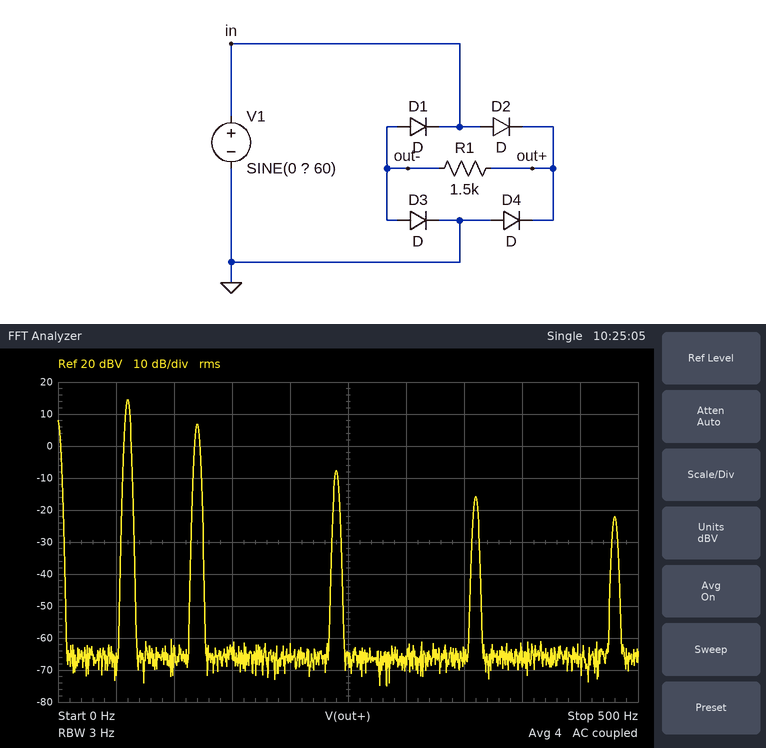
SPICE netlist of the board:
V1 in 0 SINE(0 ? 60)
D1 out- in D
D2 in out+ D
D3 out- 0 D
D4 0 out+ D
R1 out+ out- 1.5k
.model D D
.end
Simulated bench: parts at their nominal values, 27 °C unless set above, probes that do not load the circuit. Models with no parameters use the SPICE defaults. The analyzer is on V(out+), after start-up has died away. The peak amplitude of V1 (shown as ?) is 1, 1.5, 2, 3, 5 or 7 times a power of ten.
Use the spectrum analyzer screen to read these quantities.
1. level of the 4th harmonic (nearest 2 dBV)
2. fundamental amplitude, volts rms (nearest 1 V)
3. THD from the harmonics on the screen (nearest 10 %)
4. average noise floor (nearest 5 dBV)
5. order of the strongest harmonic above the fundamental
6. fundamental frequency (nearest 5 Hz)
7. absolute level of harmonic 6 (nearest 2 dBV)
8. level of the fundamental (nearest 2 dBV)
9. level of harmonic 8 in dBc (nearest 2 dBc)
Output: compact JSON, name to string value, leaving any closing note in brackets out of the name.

{"level of the 4th harmonic": "-8 dBV", "fundamental amplitude, volts rms": "5 V", "THD from the harmonics on the screen": "40 %", "average noise floor": "-65 dBV", "order of the strongest harmonic above the fundamental": "2", "fundamental frequency": "60 Hz", "absolute level of harmonic 6": "-16 dBV", "level of the fundamental": "14 dBV", "level of harmonic 8 in dBc": "-36 dBc"}
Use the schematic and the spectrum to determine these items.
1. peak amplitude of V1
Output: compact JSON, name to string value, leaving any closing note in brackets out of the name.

{"peak amplitude of V1": "15 V"}
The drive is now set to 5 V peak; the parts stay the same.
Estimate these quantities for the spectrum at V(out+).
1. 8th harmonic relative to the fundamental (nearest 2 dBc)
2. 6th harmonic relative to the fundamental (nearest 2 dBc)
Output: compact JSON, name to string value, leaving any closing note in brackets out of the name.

{"8th harmonic relative to the fundamental": "-44 dBc", "6th harmonic relative to the fundamental": "-50 dBc"}
